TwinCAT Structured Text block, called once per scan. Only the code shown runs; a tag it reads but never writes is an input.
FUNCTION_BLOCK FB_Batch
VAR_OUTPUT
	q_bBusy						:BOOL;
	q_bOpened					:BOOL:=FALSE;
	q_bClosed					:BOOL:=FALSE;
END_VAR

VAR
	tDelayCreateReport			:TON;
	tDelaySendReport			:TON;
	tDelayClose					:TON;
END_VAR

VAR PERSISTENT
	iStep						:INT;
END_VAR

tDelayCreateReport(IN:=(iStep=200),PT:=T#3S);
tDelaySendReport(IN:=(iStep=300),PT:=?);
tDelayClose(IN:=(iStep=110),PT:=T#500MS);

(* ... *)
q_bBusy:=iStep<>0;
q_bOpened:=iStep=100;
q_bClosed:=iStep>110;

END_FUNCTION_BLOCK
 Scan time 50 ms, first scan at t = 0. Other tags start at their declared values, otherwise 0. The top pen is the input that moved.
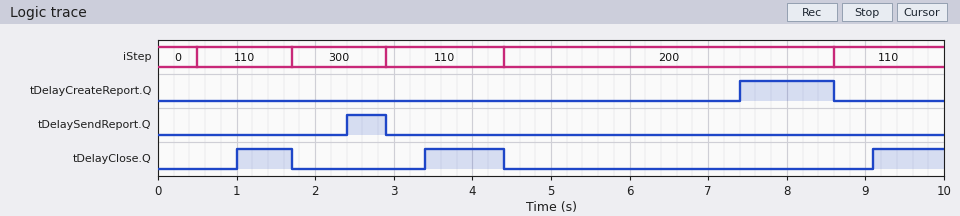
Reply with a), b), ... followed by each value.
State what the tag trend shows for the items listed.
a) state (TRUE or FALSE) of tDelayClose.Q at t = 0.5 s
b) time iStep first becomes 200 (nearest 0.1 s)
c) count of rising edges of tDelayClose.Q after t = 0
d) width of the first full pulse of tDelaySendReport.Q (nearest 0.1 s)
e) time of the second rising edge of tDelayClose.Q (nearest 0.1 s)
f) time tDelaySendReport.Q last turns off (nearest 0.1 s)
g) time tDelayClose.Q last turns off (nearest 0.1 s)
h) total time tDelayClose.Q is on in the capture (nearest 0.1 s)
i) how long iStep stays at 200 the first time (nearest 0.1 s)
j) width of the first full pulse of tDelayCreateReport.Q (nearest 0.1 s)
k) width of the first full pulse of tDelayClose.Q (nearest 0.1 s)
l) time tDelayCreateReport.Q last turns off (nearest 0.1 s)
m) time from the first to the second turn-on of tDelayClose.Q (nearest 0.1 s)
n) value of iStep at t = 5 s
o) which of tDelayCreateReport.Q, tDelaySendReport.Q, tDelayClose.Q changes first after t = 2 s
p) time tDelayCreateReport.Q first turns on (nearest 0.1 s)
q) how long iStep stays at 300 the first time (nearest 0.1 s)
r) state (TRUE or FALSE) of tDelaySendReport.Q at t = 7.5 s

a) FALSE
b) 4.4 s
c) 3
d) 0.5 s
e) 3.4 s
f) 2.9 s
g) 4.4 s
h) 2.6 s
i) 4.2 s
j) 1.2 s
k) 0.7 s
l) 8.6 s
m) 2.4 s
n) 200
o) tDelaySendReport.Q
p) 7.4 s
q) 1.2 s
r) FALSE
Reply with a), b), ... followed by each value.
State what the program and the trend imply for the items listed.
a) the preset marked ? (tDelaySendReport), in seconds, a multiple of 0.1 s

a) 0.7 s
